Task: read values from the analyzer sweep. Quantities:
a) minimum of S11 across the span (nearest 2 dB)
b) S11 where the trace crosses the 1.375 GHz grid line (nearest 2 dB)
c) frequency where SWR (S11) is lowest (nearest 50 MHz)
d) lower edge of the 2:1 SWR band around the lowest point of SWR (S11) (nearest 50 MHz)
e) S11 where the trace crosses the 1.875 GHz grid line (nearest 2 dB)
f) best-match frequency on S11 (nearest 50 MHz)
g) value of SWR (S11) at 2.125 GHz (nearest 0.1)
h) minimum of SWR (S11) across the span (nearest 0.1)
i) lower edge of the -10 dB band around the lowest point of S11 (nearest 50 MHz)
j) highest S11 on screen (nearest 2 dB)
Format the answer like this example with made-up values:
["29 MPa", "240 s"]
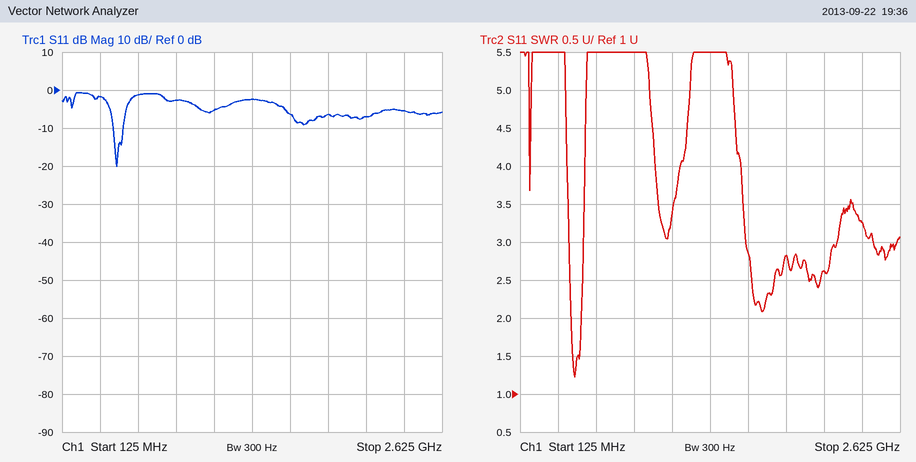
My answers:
["-20 dB", "-2 dB", "500 MHz", "450 MHz", "-6 dB", "500 MHz", "2.6", "1.2", "450 MHz", "0 dB"]
